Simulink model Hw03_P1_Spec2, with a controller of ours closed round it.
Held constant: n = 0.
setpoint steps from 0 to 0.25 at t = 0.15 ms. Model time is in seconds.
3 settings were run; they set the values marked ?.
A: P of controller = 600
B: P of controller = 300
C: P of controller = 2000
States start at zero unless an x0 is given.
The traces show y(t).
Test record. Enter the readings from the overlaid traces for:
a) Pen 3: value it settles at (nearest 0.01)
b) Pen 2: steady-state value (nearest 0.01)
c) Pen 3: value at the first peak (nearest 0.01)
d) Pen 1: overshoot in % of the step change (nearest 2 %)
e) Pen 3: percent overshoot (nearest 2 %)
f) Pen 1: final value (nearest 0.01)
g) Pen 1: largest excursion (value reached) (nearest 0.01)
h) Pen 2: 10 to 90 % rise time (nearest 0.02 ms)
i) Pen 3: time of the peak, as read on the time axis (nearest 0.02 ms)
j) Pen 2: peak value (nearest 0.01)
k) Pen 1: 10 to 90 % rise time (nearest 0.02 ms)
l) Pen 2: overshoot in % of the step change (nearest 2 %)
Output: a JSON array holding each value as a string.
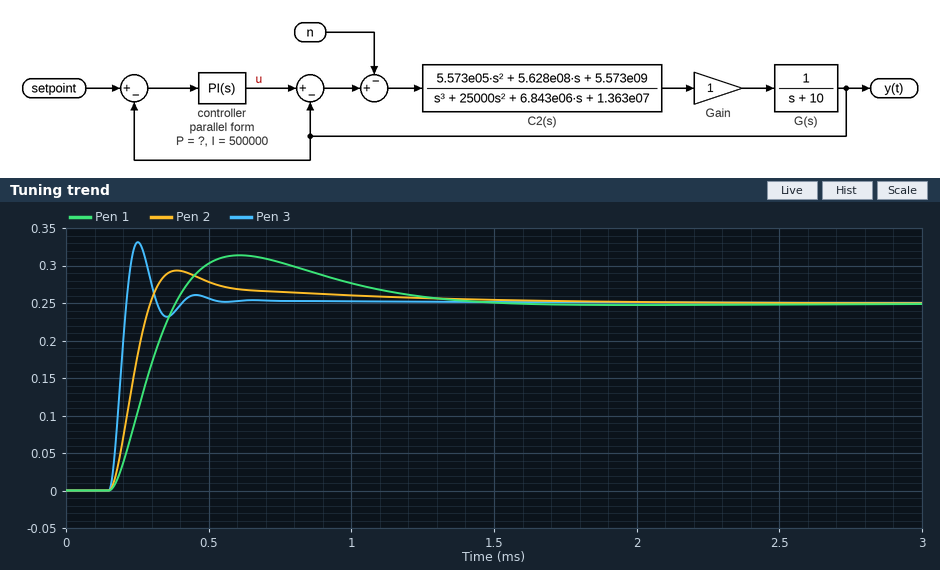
["0.25", "0.25", "0.33", "26 %", "32 %", "0.25", "0.31", "0.10 ms", "0.26 ms", "0.29", "0.16 ms", "18 %"]
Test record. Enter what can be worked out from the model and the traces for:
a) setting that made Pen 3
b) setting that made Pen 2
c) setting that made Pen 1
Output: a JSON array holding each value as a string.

["C", "A", "B"]
